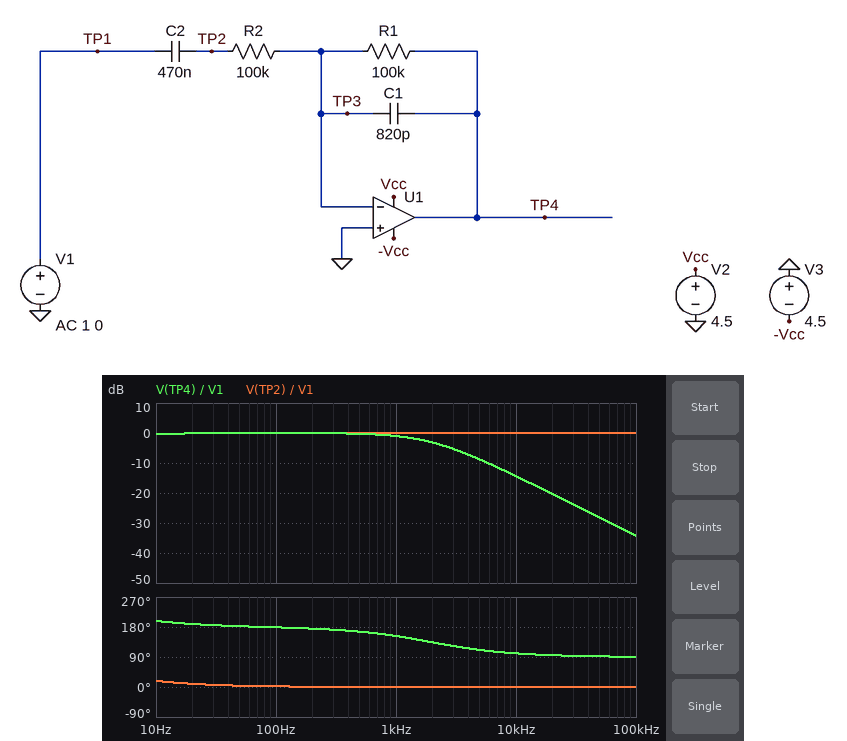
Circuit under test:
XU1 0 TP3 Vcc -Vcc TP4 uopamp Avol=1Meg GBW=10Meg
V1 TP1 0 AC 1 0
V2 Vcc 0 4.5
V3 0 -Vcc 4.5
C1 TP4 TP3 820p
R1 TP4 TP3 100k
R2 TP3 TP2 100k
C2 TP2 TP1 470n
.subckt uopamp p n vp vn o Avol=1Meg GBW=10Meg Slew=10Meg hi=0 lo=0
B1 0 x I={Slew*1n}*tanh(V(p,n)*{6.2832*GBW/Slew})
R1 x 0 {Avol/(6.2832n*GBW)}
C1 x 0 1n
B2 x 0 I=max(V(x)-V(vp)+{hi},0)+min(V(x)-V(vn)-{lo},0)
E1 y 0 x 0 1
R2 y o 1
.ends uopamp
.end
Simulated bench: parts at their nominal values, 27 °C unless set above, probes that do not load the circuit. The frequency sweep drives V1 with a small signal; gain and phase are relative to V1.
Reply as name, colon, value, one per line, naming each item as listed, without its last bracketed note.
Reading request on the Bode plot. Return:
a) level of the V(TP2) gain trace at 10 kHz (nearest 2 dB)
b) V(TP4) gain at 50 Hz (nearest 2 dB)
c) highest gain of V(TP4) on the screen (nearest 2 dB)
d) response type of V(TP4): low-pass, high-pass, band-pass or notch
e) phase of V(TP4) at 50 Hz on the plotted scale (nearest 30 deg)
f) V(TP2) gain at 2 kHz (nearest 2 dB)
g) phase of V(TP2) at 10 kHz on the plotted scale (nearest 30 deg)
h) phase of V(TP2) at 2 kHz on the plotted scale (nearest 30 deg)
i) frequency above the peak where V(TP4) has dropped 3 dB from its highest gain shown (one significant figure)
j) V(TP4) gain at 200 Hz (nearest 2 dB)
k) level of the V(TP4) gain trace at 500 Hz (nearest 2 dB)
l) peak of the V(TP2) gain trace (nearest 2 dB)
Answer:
level of the V(TP2) gain trace at 10 kHz: 0 dB
V(TP4) gain at 50 Hz: 0 dB
highest gain of V(TP4) on the screen: 0 dB
response type of V(TP4): low-pass, high-pass, band-pass or notch: low-pass
phase of V(TP4) at 50 Hz on the plotted scale: 180 deg
V(TP2) gain at 2 kHz: 0 dB
phase of V(TP2) at 10 kHz on the plotted scale: 0 deg
phase of V(TP2) at 2 kHz on the plotted scale: 0 deg
frequency above the peak where V(TP4) has dropped 3 dB from its highest gain shown: 2 kHz
V(TP4) gain at 200 Hz: 0 dB
level of the V(TP4) gain trace at 500 Hz: 0 dB
peak of the V(TP2) gain trace: 0 dB
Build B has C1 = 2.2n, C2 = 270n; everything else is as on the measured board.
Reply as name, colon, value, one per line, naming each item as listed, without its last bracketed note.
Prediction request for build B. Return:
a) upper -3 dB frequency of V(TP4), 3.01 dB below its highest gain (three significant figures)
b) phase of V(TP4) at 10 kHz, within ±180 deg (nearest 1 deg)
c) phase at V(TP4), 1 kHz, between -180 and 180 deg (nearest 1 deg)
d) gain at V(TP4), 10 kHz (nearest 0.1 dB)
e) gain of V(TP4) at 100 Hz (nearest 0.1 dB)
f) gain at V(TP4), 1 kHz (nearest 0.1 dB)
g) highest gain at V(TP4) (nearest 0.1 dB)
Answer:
upper -3 dB frequency of V(TP4), 3.01 dB below its highest gain: 735 Hz
phase of V(TP4) at 10 kHz, within ±180 deg: 94 deg
phase at V(TP4), 1 kHz, between -180 and 180 deg: 126 deg
gain at V(TP4), 10 kHz: -22.8 dB
gain of V(TP4) at 100 Hz: -0.1 dB
gain at V(TP4), 1 kHz: -4.6 dB
highest gain at V(TP4): -0.1 dB
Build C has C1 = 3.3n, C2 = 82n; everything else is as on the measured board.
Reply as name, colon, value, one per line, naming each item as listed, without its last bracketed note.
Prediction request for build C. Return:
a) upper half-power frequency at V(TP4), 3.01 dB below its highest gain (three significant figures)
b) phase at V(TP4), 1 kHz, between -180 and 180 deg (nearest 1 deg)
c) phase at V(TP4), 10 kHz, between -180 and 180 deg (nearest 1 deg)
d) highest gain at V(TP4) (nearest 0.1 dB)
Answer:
upper half-power frequency at V(TP4), 3.01 dB below its highest gain: 520 Hz
phase at V(TP4), 1 kHz, between -180 and 180 deg: 117 deg
phase at V(TP4), 10 kHz, between -180 and 180 deg: 93 deg
highest gain at V(TP4): -0.3 dB
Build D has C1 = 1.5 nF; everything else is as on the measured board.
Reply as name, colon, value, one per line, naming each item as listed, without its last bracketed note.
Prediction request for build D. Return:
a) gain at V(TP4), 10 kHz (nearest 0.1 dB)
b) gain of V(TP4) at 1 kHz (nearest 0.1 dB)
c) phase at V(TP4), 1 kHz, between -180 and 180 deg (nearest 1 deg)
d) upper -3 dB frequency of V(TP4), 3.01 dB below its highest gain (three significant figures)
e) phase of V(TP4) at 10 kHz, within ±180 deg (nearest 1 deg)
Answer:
gain at V(TP4), 10 kHz: -19.5 dB
gain of V(TP4) at 1 kHz: -2.8 dB
phase at V(TP4), 1 kHz, between -180 and 180 deg: 137 deg
upper -3 dB frequency of V(TP4), 3.01 dB below its highest gain: 1.07 kHz
phase of V(TP4) at 10 kHz, within ±180 deg: 96 deg
